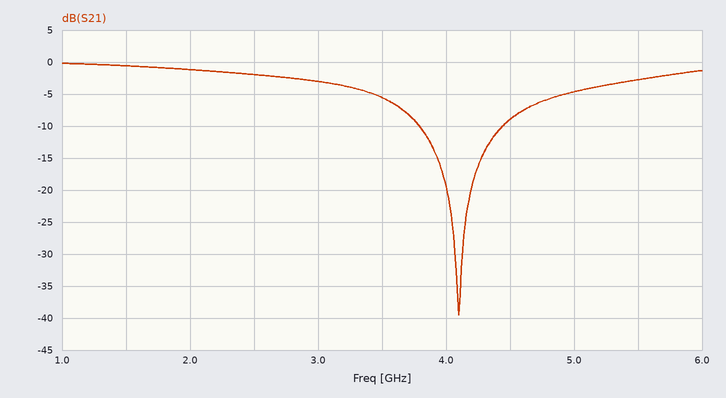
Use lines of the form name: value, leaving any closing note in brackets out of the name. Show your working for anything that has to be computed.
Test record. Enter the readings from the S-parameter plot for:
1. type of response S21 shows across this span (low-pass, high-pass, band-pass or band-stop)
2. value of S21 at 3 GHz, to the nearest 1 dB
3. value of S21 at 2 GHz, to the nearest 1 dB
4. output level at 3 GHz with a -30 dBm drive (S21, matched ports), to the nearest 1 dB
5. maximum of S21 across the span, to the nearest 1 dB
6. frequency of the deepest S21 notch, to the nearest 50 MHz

type of response S21 shows across this span: band-stop
value of S21 at 3 GHz, to the nearest 1 dB: -3 dB
value of S21 at 2 GHz, to the nearest 1 dB: -1 dB
output level at 3 GHz with a -30 dBm drive (S21, matched ports), to the nearest 1 dB: -30 dBm + (-3 dB) = -33 dBm
maximum of S21 across the span, to the nearest 1 dB: 0 dB
frequency of the deepest S21 notch, to the nearest 50 MHz: 4.10 GHz
